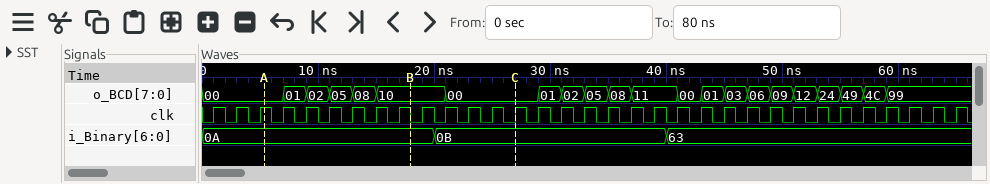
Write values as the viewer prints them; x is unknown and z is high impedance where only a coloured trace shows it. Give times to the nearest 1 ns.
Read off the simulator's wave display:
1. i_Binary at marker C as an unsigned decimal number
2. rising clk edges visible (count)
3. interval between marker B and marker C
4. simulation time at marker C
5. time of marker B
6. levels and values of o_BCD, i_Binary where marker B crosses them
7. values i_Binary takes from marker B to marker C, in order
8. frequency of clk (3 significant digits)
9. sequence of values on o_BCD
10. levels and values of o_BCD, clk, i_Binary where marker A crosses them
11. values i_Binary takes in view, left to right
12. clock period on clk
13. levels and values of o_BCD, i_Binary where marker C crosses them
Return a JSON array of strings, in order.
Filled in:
["11", "33", "9 ns", "27 ns", "18 ns", "o_BCD=10, i_Binary=0A", "0A, 0B", "500 MHz", "00, 01, 02, 05, 08, 10, 00, 01, 02, 05, 08, 11, 00, 01, 03, 06, 09, 12, 24, 49, 4C, 99", "o_BCD=00, clk=1, i_Binary=0A", "0A, 0B, 63", "2 ns", "o_BCD=00, i_Binary=0B"]
